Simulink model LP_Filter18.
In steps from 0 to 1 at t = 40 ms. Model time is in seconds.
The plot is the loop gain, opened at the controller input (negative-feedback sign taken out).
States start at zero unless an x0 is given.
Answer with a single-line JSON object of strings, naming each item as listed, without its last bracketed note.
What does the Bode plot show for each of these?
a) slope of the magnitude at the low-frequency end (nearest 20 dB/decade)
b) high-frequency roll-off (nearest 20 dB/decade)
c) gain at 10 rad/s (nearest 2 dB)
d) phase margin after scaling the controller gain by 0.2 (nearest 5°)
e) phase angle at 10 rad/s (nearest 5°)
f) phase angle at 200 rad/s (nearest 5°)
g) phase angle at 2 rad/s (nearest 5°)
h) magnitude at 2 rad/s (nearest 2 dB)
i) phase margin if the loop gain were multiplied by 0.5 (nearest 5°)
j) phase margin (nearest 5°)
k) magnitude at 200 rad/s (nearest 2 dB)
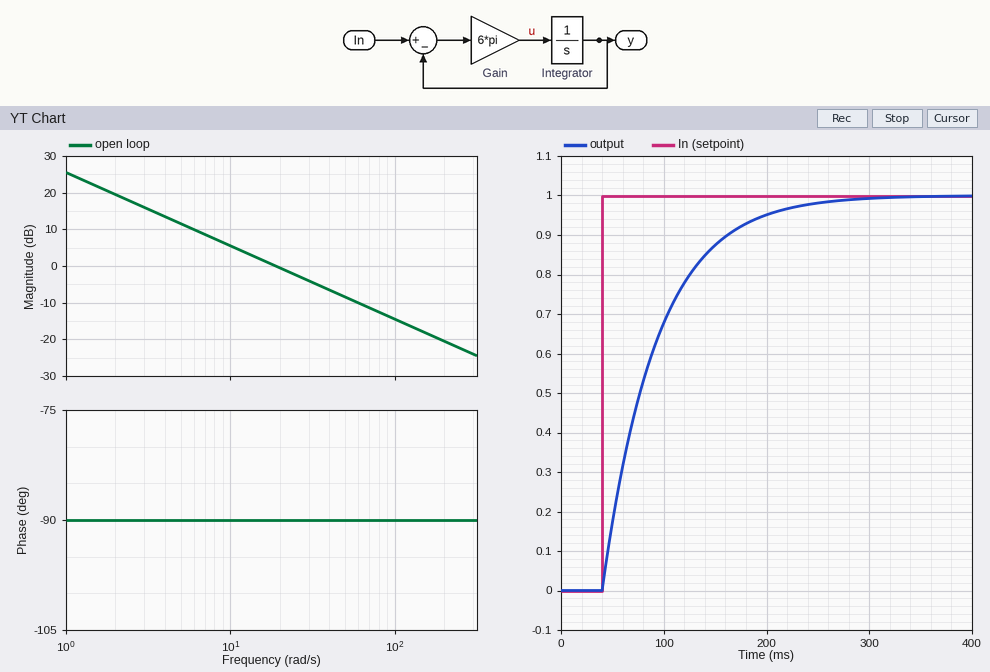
{"slope of the magnitude at the low-frequency end": "-20 dB/decade", "high-frequency roll-off": "-20 dB/decade", "gain at 10 rad/s": "6 dB", "phase margin after scaling the controller gain by 0.2": "90°", "phase angle at 10 rad/s": "-90°", "phase angle at 200 rad/s": "-90°", "phase angle at 2 rad/s": "-90°", "magnitude at 2 rad/s": "20 dB", "phase margin if the loop gain were multiplied by 0.5": "90°", "phase margin": "90°", "magnitude at 200 rad/s": "-20 dB"}
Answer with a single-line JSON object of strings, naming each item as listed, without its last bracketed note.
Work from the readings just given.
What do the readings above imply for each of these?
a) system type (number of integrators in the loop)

{"system type": "1"}
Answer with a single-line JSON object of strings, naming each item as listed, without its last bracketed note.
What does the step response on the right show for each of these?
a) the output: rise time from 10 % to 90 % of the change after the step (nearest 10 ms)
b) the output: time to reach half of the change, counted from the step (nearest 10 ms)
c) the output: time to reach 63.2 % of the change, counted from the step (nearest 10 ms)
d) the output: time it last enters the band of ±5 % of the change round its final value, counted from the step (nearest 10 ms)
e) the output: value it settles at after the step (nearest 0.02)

{"the output: rise time from 10 % to 90 % of the change after the step": "120 ms", "the output: time to reach half of the change, counted from the step": "40 ms", "the output: time to reach 63.2 % of the change, counted from the step": "50 ms", "the output: time it last enters the band of ±5 % of the change round its final value, counted from the step": "160 ms", "the output: value it settles at after the step": "1.00"}
